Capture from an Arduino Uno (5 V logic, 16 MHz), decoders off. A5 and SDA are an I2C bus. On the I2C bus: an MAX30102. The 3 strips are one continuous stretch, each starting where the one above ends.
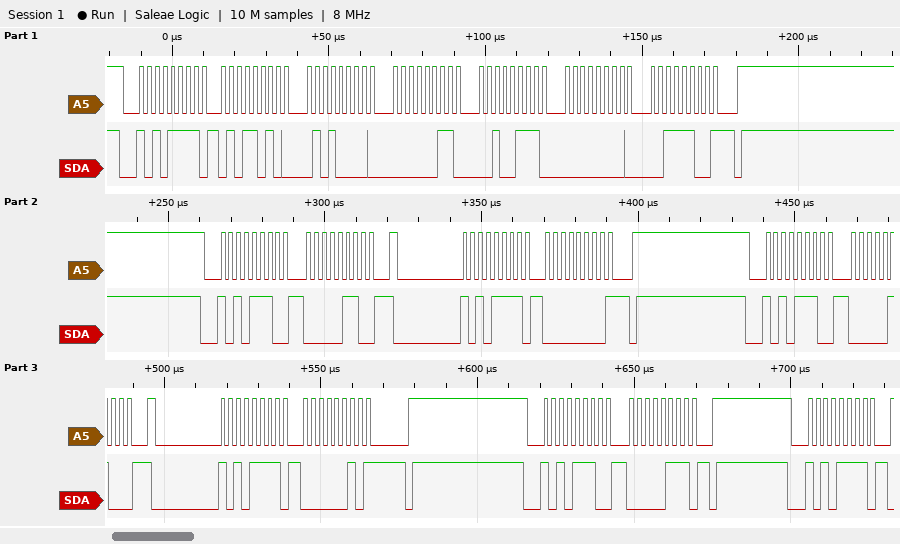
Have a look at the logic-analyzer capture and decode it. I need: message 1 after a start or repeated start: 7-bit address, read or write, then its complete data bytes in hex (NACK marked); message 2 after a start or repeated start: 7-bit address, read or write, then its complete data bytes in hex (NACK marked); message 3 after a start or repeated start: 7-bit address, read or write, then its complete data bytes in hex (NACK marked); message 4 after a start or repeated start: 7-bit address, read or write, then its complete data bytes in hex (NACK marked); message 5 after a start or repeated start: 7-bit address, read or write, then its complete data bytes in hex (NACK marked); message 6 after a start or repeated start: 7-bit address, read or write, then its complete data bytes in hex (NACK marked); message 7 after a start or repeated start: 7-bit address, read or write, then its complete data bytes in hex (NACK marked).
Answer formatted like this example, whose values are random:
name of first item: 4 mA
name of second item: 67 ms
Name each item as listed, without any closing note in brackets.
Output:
message 1 after a start or repeated start: 7-bit address, read or write, then its complete data bytes in hex: 0x57 read: 5A 50 03 27 00 3C NACK
message 2 after a start or repeated start: 7-bit address, read or write, then its complete data bytes in hex: 0x57 write: 06
message 3 after a start or repeated start: 7-bit address, read or write, then its complete data bytes in hex: 0x57 read: 00 NACK
message 4 after a start or repeated start: 7-bit address, read or write, then its complete data bytes in hex: 0x57 write: 04
message 5 after a start or repeated start: 7-bit address, read or write, then its complete data bytes in hex: 0x57 read: 02 NACK
message 6 after a start or repeated start: 7-bit address, read or write, then its complete data bytes in hex: 0x57 write: 07
message 7 after a start or repeated start: 7-bit address, read or write, then its complete data bytes in hex: 0x57 read
